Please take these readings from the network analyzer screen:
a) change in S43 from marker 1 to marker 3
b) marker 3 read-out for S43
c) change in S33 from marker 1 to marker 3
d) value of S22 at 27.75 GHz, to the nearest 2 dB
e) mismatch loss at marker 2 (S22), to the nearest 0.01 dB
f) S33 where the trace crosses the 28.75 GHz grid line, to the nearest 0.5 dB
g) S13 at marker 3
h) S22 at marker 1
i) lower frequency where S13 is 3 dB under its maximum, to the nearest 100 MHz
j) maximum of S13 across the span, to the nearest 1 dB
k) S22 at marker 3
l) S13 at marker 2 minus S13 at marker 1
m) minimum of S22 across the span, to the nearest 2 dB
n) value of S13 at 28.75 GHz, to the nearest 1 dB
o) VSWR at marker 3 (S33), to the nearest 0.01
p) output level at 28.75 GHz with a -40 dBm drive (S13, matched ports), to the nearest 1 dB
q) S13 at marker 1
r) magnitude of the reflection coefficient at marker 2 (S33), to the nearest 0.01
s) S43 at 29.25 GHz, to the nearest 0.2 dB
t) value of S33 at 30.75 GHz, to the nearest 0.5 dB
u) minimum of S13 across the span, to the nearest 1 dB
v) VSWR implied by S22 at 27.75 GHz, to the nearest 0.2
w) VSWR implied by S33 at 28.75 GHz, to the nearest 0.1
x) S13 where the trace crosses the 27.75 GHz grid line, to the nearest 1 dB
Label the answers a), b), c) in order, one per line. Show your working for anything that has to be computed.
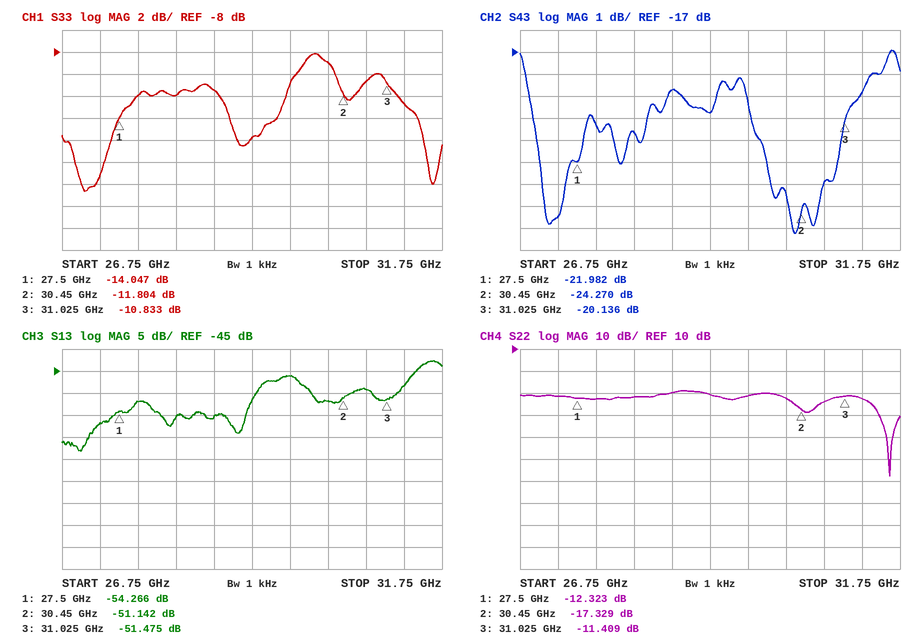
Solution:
a) -20.136 − (-21.982) = 1.846 dB
b) -20.136 dB
c) -10.833 − (-14.047) = 3.214 dB
d) -12 dB
e) −10 log10(1 − 10^(-17.329/10)) ≈ 0.08 dB
f) -11.5 dB
g) -51.475 dB
h) -12.323 dB
i) 31.4 GHz
j) -43 dB
k) -11.409 dB
l) -51.142 − (-54.266) = 3.124 dB
m) -48 dB
n) -55 dB
o) (1 + 0.2873)/(1 − 0.2873) ≈ 1.81
p) -40 dBm + (-55 dB) = -95 dBm
q) -54.266 dB
r) 10^(-11.804/20) ≈ 0.26
s) -19.8 dB
t) -10.5 dB
u) -63 dB
v) |Γ| = 10^(-12/20) = 0.2512; VSWR = (1 + 0.2512)/(1 − 0.2512) ≈ 1.67, so 1.6 to the nearest 0.2
w) |Γ| = 10^(-11.5/20) = 0.2661; VSWR = (1 + 0.2661)/(1 − 0.2661) ≈ 1.7
x) -52 dB
